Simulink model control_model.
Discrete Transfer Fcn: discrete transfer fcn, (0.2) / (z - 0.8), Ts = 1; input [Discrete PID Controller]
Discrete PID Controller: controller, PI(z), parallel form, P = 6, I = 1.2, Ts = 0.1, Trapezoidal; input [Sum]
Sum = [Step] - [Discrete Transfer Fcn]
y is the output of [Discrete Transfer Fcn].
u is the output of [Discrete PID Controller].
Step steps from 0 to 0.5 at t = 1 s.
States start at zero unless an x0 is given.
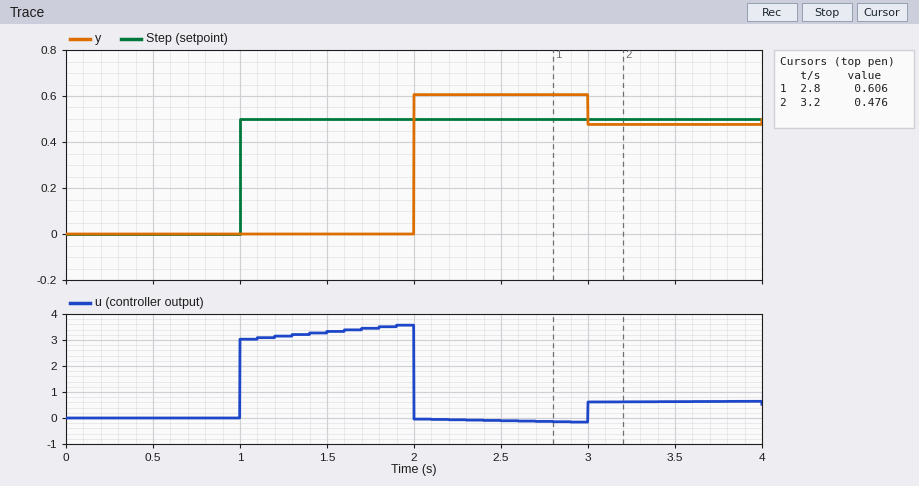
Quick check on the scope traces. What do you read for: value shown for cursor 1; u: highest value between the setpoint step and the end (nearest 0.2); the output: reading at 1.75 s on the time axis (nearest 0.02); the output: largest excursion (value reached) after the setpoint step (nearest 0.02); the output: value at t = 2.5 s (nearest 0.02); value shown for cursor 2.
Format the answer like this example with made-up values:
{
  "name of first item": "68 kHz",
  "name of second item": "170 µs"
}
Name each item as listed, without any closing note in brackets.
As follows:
{
  "value shown for cursor 1": "0.606",
  "u: highest value between the setpoint step and the end": "3.6",
  "the output: reading at 1.75 s on the time axis": "0.00",
  "the output: largest excursion (value reached) after the setpoint step": "0.60",
  "the output: value at t = 2.5 s": "0.60",
  "value shown for cursor 2": "0.476"
}
